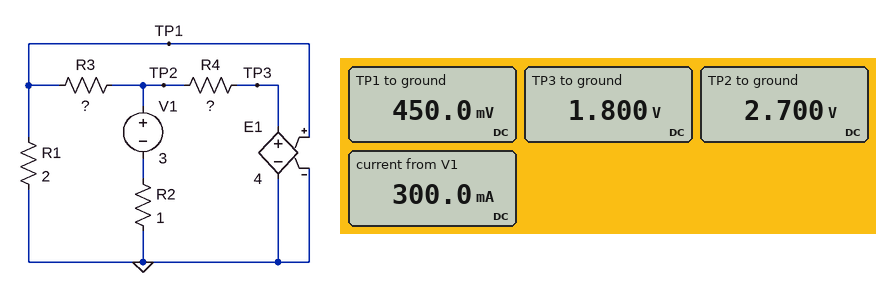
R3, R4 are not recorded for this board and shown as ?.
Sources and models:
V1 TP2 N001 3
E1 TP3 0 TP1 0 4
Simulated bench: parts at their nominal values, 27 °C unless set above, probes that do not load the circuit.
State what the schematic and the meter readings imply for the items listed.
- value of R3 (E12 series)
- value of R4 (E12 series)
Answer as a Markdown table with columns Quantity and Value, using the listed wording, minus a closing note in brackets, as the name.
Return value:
| Quantity | Value |
|---|---|
| value of R3 | 10 Ω |
| value of R4 | 12 Ω |
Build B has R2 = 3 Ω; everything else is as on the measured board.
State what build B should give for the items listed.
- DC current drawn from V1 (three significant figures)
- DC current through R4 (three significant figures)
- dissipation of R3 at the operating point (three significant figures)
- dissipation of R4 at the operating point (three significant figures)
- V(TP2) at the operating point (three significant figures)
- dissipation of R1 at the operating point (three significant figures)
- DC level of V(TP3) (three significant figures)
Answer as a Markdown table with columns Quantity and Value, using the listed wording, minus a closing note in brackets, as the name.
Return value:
| Quantity | Value |
|---|---|
| DC current drawn from V1 | 250 mA |
| DC current through R4 | 62.5 mA |
| dissipation of R3 at the operating point | 352 mW |
| dissipation of R4 at the operating point | 46.9 mW |
| V(TP2) at the operating point | 2.25 V |
| dissipation of R1 at the operating point | 70.3 mW |
| DC level of V(TP3) | 1.50 V |
